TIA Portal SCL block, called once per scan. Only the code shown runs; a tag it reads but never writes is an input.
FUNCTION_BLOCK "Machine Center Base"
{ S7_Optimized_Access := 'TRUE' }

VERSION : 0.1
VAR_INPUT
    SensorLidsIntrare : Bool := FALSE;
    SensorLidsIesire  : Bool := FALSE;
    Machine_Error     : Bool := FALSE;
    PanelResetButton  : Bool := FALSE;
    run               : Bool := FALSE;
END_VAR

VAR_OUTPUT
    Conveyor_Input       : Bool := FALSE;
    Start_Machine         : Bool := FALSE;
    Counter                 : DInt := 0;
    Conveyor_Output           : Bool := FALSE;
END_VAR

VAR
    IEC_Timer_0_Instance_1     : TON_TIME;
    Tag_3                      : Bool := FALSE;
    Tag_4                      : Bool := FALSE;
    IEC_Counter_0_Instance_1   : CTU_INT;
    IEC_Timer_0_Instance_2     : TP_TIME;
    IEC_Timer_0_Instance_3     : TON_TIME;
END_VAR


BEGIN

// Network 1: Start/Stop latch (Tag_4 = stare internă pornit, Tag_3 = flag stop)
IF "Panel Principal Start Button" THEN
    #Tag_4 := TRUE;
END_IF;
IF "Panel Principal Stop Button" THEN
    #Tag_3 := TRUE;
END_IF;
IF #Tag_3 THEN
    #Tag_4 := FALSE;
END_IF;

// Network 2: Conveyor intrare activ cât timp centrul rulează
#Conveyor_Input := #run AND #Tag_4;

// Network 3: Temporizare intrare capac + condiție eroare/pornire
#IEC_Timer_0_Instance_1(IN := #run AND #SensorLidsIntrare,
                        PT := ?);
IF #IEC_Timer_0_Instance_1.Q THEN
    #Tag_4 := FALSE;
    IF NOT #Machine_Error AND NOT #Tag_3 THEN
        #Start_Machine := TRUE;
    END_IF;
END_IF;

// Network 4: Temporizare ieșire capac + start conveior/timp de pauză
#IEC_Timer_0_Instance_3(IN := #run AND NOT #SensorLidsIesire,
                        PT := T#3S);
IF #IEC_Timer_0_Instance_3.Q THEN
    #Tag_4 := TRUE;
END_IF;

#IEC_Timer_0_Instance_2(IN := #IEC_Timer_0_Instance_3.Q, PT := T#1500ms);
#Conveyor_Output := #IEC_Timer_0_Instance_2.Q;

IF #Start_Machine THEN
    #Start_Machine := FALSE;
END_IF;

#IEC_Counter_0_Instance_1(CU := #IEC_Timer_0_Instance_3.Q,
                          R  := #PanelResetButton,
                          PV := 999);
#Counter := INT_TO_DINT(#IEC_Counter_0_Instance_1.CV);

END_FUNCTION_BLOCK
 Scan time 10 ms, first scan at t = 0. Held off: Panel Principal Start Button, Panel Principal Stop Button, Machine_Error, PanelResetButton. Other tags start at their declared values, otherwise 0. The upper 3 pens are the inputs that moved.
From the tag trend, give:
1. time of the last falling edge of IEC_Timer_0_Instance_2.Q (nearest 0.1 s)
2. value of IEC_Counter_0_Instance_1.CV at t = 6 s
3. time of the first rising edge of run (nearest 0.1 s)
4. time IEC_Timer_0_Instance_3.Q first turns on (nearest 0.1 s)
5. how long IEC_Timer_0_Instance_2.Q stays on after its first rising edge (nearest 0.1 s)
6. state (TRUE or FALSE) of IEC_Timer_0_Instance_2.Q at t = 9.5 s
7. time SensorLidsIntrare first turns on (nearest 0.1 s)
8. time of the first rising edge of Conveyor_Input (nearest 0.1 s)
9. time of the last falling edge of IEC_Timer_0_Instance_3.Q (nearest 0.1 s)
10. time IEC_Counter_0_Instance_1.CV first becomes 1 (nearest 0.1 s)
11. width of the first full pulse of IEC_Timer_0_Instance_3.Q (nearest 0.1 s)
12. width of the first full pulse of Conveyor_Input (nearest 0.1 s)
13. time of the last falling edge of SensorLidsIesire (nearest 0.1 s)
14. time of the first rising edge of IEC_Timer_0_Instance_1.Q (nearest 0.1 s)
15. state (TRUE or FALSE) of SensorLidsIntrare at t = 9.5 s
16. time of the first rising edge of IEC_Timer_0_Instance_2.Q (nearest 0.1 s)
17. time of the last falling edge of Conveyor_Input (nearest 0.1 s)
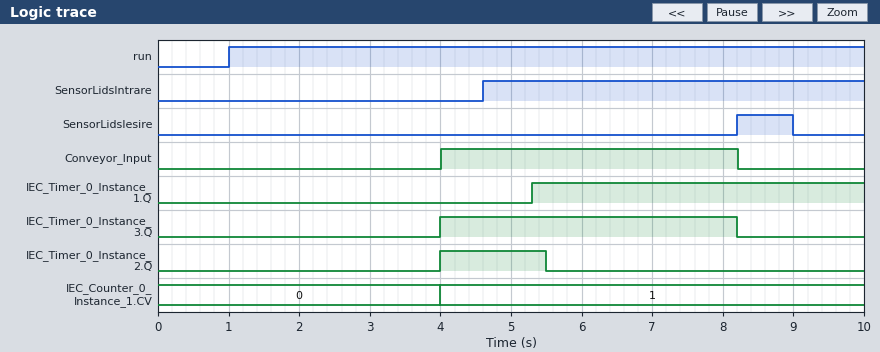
5.5 s
1
1.0 s
4.0 s
1.5 s
FALSE
4.6 s
4.0 s
8.2 s
4.0 s
4.2 s
4.2 s
9.0 s
5.3 s
TRUE
4.0 s
8.2 s
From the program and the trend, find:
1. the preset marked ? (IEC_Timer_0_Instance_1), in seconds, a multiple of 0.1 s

0.7 s
